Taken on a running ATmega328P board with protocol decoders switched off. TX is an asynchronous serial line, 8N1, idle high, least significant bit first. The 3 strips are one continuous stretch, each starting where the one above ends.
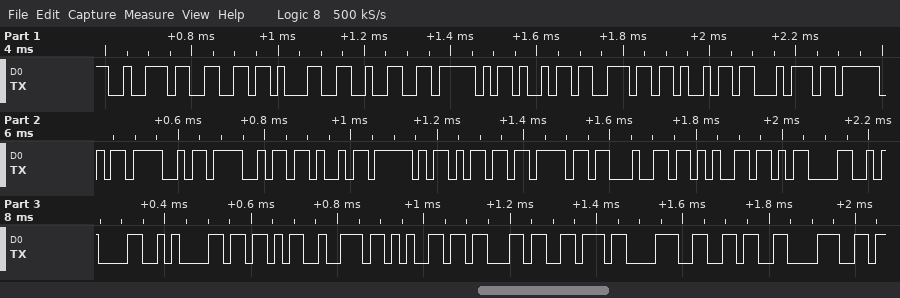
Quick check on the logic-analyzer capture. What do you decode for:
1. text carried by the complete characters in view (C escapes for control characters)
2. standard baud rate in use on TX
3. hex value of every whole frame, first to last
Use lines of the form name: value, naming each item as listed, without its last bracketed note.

text carried by the complete characters in view: "rf12_init_OOK_mode\r\n\n[recv868"
standard baud rate in use on TX: 57600 baud
hex value of every whole frame, first to last: 0x72 0x66 0x31 0x32 0x5F 0x69 0x6E 0x69 0x74 0x5F 0x4F 0x4F 0x4B 0x5F 0x6D 0x6F 0x64 0x65 0x0D 0x0A 0x0A 0x5B 0x72 0x65 0x63 0x76 0x38 0x36 0x38
